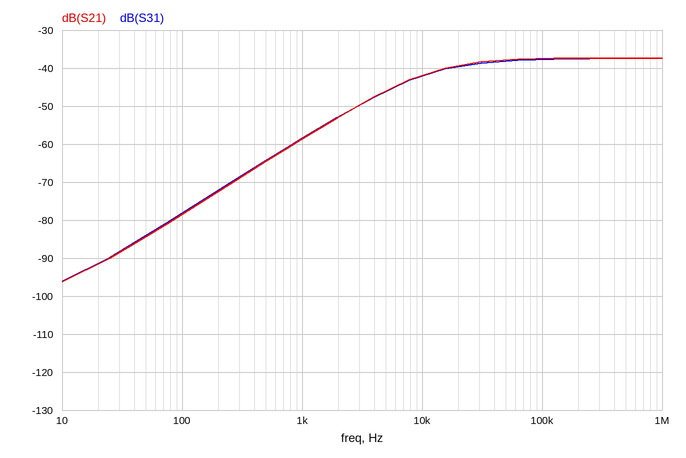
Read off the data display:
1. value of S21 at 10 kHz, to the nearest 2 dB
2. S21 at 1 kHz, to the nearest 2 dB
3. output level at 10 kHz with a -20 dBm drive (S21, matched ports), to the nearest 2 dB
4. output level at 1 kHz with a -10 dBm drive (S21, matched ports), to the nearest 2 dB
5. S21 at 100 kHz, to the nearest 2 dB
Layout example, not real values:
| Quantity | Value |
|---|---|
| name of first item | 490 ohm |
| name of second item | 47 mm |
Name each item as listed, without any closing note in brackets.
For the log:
| Quantity | Value |
|---|---|
| value of S21 at 10 kHz, to the nearest 2 dB | -42 dB |
| S21 at 1 kHz, to the nearest 2 dB | -58 dB |
| output level at 10 kHz with a -20 dBm drive (S21, matched ports), to the nearest 2 dB | -62 dBm |
| output level at 1 kHz with a -10 dBm drive (S21, matched ports), to the nearest 2 dB | -68 dBm |
| S21 at 100 kHz, to the nearest 2 dB | -38 dB |
